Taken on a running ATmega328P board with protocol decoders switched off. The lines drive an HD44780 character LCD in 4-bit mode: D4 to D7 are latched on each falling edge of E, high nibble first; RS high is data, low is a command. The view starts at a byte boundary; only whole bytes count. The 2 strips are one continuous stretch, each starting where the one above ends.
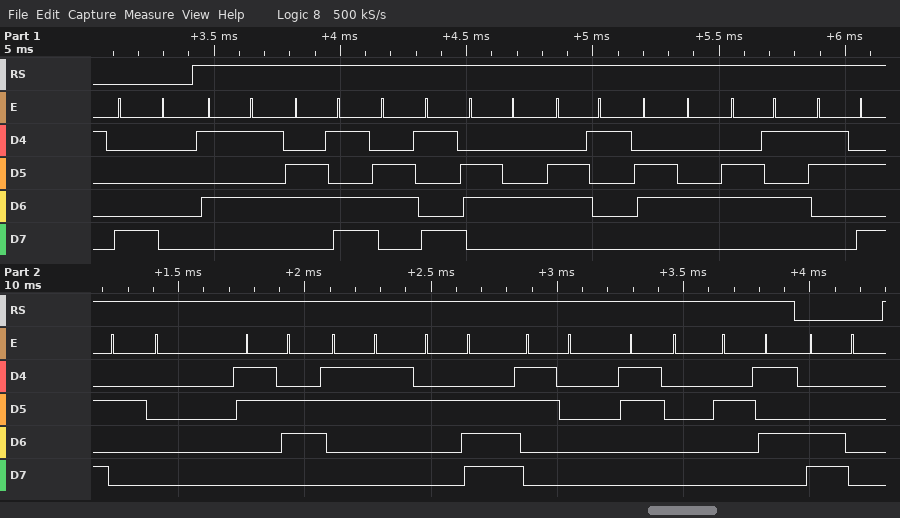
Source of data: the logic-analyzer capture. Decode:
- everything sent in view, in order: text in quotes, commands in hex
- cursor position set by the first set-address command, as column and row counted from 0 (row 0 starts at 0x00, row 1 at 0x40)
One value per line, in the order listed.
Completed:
0x80 "Umidade: 63.00%" 0xC0
column 0, row 0
